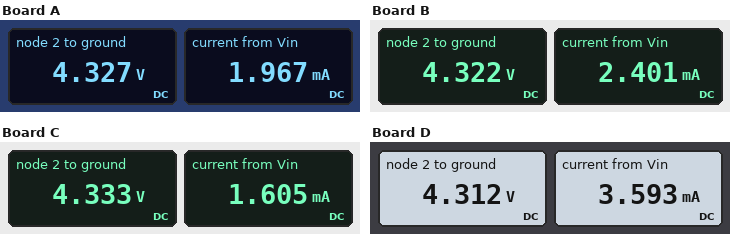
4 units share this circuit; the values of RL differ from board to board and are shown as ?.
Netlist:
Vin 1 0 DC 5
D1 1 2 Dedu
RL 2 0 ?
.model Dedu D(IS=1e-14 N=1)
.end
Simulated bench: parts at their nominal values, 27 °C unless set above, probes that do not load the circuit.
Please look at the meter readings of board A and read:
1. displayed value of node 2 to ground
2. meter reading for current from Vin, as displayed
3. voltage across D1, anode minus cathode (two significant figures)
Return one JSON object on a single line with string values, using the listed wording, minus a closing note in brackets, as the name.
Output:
{"displayed value of node 2 to ground": "4.327 V", "meter reading for current from Vin, as displayed": "1.967 mA", "voltage across D1, anode minus cathode": "670 mV"}
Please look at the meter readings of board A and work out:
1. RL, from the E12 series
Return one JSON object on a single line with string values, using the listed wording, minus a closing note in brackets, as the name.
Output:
{"RL, from the E12 series": "2.2 kΩ"}
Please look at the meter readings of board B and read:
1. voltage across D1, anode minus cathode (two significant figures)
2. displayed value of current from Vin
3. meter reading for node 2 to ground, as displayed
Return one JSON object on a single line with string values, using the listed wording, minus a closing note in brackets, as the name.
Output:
{"voltage across D1, anode minus cathode": "680 mV", "displayed value of current from Vin": "2.401 mA", "meter reading for node 2 to ground, as displayed": "4.322 V"}
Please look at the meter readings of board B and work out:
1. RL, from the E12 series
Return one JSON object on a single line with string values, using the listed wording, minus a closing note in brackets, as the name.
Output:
{"RL, from the E12 series": "1.8 kΩ"}
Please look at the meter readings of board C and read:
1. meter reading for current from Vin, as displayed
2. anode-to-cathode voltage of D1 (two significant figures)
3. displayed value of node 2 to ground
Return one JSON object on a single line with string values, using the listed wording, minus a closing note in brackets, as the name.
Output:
{"meter reading for current from Vin, as displayed": "1.605 mA", "anode-to-cathode voltage of D1": "670 mV", "displayed value of node 2 to ground": "4.333 V"}
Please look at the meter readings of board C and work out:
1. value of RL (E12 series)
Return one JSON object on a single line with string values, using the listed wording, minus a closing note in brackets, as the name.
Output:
{"value of RL": "2.7 kΩ"}
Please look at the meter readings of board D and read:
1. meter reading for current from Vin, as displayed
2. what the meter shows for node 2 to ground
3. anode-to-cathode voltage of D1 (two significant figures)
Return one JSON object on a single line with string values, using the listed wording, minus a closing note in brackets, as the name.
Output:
{"meter reading for current from Vin, as displayed": "3.593 mA", "what the meter shows for node 2 to ground": "4.312 V", "anode-to-cathode voltage of D1": "690 mV"}
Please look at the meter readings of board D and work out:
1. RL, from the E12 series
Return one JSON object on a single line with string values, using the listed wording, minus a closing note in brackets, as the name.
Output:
{"RL, from the E12 series": "1.2 kΩ"}
